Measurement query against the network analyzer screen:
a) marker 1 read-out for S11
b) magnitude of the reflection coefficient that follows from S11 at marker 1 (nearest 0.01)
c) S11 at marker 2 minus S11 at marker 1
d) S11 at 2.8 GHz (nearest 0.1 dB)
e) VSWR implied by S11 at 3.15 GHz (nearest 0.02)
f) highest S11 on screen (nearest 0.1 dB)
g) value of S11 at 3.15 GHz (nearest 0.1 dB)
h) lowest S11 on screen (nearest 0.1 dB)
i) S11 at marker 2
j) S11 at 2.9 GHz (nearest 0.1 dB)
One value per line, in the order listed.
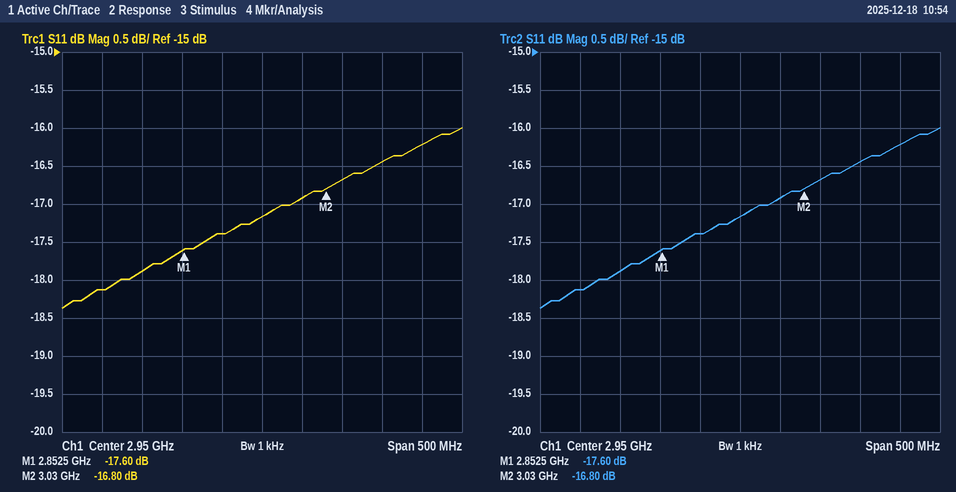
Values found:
-17.60 dB
0.13
0.80 dB
-17.9 dB
1.36
-16.0 dB
-16.2 dB
-18.4 dB
-16.80 dB
-17.4 dB
